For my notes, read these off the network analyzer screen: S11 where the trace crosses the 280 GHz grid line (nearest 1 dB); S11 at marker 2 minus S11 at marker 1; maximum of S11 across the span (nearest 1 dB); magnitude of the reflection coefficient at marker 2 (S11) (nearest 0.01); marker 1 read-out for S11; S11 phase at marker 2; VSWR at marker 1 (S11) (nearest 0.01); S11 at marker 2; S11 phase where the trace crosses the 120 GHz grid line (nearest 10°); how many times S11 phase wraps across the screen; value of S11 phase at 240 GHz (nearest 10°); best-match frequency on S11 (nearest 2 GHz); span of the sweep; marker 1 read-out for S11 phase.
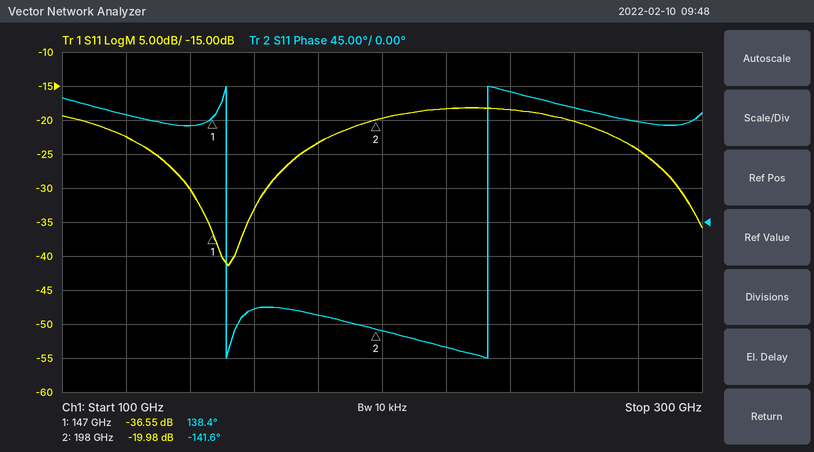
-24 dB
16.57 dB
-18 dB
0.10
-36.55 dB
-141.6°
1.03
-19.98 dB
140°
2
170°
152 GHz
200 GHz
138.4°
